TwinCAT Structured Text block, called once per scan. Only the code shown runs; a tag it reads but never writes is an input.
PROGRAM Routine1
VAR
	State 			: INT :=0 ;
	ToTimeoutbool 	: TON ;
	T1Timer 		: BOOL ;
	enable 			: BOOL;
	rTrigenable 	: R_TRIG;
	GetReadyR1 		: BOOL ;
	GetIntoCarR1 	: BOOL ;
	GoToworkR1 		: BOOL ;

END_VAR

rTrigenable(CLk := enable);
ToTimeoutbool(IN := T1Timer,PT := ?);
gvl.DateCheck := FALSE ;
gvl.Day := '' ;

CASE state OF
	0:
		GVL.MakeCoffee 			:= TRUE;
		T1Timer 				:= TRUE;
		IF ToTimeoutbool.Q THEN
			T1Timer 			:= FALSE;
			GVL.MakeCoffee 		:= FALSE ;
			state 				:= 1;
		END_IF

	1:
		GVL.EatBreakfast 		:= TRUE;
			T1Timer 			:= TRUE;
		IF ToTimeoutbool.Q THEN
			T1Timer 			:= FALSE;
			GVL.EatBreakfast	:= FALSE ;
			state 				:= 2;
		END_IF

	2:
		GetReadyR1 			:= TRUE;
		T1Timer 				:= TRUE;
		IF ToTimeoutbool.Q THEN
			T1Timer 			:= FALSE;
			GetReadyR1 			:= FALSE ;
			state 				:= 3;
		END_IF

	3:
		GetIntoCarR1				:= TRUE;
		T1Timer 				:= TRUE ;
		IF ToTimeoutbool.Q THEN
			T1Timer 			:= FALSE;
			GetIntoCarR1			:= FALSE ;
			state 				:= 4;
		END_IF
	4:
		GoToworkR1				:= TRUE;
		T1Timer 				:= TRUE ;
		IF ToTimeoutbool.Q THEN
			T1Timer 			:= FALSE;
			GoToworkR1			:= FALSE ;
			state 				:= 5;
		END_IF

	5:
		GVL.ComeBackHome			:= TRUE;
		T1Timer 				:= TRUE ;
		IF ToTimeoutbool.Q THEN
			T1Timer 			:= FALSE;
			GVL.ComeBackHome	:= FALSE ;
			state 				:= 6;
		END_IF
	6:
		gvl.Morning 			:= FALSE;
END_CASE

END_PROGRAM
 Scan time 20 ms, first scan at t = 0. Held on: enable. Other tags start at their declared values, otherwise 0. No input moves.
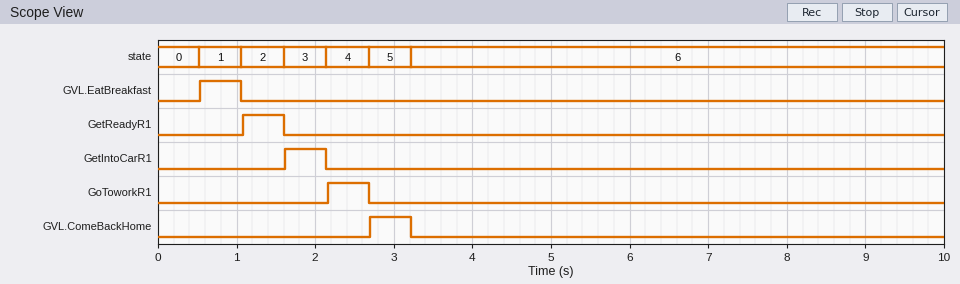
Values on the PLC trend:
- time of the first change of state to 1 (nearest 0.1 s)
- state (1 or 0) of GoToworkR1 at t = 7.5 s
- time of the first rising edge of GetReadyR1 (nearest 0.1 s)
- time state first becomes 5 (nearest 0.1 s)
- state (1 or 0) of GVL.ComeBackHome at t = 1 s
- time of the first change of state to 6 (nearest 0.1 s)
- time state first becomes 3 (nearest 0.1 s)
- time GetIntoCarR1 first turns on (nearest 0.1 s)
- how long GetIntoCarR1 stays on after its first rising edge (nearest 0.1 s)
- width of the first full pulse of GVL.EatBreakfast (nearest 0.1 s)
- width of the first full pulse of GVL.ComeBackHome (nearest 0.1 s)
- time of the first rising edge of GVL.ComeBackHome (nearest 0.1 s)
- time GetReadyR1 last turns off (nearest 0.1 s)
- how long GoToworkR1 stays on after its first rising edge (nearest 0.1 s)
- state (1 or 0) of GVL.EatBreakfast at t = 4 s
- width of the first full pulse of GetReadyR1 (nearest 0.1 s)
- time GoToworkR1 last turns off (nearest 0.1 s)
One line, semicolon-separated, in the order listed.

0.5 s; 0; 1.1 s; 2.7 s; 0; 3.2 s; 1.6 s; 1.6 s; 0.5 s; 0.5 s; 0.5 s; 2.7 s; 1.6 s; 0.5 s; 0; 0.5 s; 2.7 s
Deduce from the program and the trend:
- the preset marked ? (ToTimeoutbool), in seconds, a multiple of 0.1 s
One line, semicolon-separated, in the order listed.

0.5 s
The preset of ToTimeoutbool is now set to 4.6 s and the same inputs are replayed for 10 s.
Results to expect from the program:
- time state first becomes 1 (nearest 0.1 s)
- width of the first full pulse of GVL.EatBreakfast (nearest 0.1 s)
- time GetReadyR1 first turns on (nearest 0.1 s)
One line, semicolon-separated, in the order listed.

4.6 s; 4.6 s; 9.3 s
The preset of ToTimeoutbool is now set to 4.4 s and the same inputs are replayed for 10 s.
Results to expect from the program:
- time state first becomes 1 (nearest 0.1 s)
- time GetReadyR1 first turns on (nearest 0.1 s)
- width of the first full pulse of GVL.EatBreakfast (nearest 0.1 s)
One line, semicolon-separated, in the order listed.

4.4 s; 8.9 s; 4.4 s
